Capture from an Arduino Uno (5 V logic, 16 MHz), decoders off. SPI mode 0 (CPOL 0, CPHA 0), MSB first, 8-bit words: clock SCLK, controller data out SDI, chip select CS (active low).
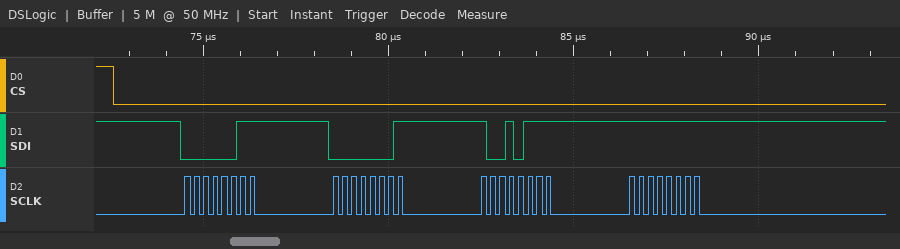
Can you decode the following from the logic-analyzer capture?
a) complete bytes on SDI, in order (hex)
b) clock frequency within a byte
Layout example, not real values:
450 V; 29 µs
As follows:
0x03 0x01 0x97 0xFF; 4 MHz
